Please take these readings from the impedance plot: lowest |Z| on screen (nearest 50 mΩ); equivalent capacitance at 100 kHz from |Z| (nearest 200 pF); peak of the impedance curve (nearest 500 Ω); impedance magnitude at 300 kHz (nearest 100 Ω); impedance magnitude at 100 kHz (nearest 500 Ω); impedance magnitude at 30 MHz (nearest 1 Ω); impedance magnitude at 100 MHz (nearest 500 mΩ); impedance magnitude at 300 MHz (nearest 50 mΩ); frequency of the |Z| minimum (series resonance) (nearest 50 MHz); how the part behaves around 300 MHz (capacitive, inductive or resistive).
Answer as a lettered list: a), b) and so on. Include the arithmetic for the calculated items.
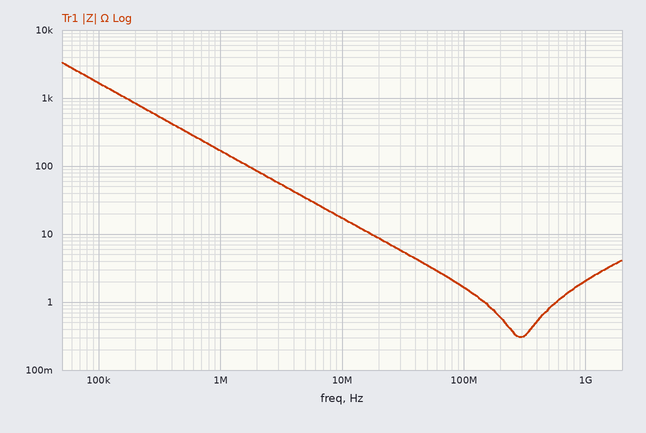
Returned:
a) 300 mΩ
b) C = 1/(2π × 100 kHz × 1.5 kΩ) ≈ 1.06 nF, so 1.0 nF to the nearest 200 pF
c) 3.5 kΩ
d) 600 Ω
e) 1.5 kΩ
f) 6 Ω
g) 1.5 Ω
h) 300 mΩ
i) 300 MHz
j) resistive
